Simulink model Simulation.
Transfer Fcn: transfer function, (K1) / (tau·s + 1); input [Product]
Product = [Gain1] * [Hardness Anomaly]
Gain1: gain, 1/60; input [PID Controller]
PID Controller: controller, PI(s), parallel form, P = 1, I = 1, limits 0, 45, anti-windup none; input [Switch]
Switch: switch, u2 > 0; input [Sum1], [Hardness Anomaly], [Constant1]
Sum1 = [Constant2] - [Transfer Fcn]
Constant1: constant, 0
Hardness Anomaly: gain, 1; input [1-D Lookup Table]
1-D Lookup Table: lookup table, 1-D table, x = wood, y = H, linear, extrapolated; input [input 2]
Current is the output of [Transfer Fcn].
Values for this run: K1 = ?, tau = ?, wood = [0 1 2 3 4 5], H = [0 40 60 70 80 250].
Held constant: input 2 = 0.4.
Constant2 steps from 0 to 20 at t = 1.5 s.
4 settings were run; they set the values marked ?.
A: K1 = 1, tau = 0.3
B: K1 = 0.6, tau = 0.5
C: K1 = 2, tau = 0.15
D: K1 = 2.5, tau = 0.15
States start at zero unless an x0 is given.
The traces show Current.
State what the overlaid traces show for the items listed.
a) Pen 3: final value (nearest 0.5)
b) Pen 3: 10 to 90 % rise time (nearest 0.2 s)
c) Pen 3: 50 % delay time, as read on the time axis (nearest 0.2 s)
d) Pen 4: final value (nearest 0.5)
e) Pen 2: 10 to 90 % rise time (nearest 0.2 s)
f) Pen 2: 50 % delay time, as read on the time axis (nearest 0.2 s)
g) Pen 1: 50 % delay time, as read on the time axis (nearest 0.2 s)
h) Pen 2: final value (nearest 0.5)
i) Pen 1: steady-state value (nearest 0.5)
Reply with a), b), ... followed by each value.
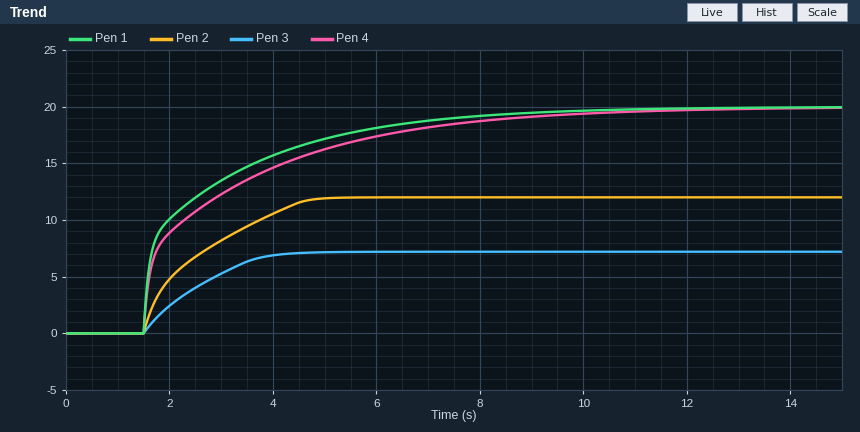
a) 7.0
b) 2.0 s
c) 2.4 s
d) 20.0
e) 2.6 s
f) 2.2 s
g) 2.0 s
h) 12.0
i) 20.0
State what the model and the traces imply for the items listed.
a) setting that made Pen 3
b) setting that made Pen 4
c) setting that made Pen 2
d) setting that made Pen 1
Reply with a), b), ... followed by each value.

a) B
b) C
c) A
d) D
